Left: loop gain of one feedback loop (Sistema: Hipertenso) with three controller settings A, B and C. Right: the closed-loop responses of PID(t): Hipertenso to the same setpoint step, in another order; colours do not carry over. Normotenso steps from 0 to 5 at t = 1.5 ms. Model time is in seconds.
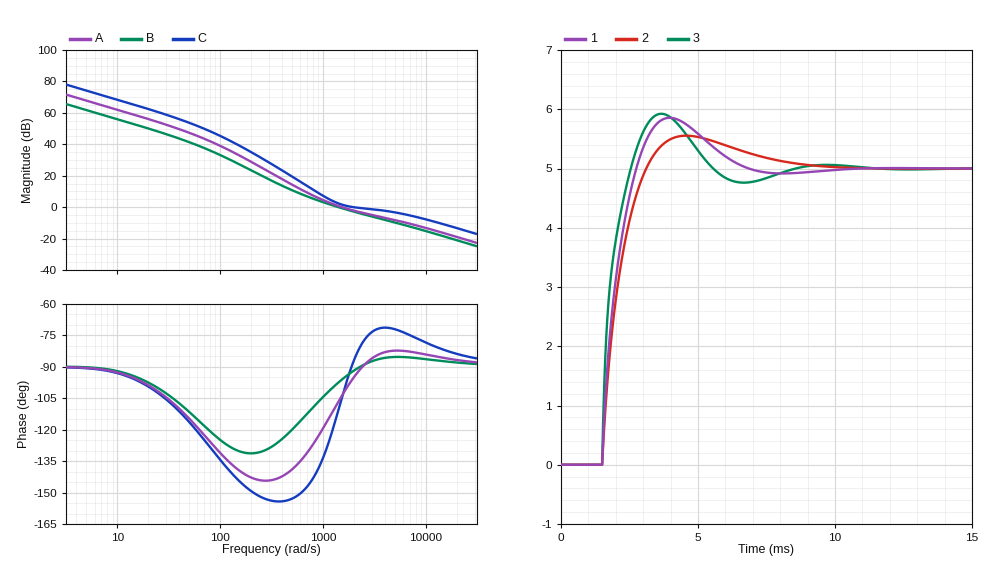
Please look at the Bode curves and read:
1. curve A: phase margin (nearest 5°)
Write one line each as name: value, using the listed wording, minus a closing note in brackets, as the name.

curve A: phase margin: 75°
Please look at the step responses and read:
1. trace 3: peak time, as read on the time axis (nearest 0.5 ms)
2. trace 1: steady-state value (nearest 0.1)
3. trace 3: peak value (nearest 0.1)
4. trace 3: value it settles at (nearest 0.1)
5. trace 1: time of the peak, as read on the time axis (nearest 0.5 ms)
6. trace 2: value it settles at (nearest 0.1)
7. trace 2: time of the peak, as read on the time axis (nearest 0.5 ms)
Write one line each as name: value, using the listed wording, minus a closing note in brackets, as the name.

trace 3: peak time, as read on the time axis: 3.5 ms
trace 1: steady-state value: 5.0
trace 3: peak value: 5.9
trace 3: value it settles at: 5.0
trace 1: time of the peak, as read on the time axis: 4.0 ms
trace 2: value it settles at: 5.0
trace 2: time of the peak, as read on the time axis: 4.5 ms
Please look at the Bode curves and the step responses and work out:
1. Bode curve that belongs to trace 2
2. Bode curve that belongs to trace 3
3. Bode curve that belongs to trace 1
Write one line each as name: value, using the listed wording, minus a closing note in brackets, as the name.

Bode curve that belongs to trace 2: B
Bode curve that belongs to trace 3: C
Bode curve that belongs to trace 1: A
